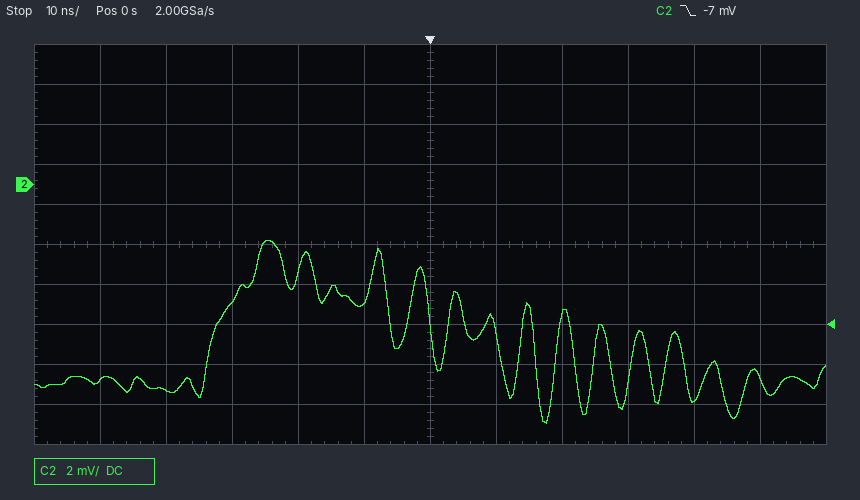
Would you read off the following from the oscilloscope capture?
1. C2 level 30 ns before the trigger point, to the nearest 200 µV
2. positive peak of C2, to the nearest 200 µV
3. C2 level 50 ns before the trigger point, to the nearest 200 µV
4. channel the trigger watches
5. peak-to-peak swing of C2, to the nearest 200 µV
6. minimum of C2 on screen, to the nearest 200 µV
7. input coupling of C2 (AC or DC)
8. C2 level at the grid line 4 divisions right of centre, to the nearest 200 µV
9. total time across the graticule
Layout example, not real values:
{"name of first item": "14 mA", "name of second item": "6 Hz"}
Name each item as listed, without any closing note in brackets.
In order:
{"C2 level 30 ns before the trigger point, to the nearest 200 µV": "-5.8 mV", "positive peak of C2, to the nearest 200 µV": "-2.8 mV", "C2 level 50 ns before the trigger point, to the nearest 200 µV": "-9.8 mV", "channel the trigger watches": "C2", "peak-to-peak swing of C2, to the nearest 200 µV": "9.2 mV", "minimum of C2 on screen, to the nearest 200 µV": "-12.0 mV", "input coupling of C2": "DC", "C2 level at the grid line 4 divisions right of centre, to the nearest 200 µV": "-10.8 mV", "total time across the graticule": "120 ns"}
